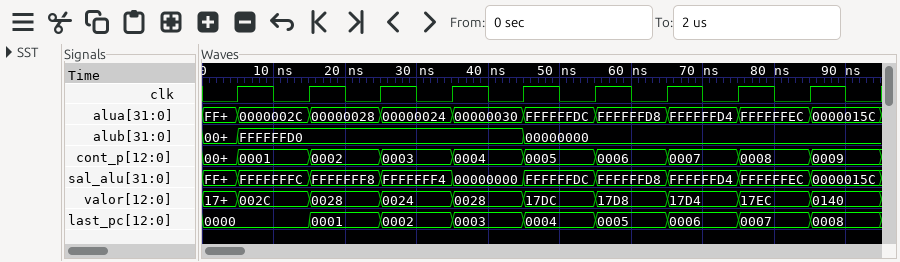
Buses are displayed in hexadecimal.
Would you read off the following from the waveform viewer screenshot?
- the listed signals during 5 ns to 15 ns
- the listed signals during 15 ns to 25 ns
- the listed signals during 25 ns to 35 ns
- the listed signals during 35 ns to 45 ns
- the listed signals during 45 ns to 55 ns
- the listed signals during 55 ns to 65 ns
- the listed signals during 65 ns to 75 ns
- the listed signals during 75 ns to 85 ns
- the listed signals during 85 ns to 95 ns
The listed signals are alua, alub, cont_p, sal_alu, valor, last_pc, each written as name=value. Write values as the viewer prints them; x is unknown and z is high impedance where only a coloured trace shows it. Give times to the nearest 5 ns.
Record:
alua=0000002C, alub=FFFFFFD0, cont_p=0001, sal_alu=FFFFFFFC, valor=002C, last_pc=0000
alua=00000028, alub=FFFFFFD0, cont_p=0002, sal_alu=FFFFFFF8, valor=0028, last_pc=0001
alua=00000024, alub=FFFFFFD0, cont_p=0003, sal_alu=FFFFFFF4, valor=0024, last_pc=0002
alua=00000030, alub=FFFFFFD0, cont_p=0004, sal_alu=00000000, valor=0028, last_pc=0003
alua=FFFFFFDC, alub=00000000, cont_p=0005, sal_alu=FFFFFFDC, valor=17DC, last_pc=0004
alua=FFFFFFD8, alub=00000000, cont_p=0006, sal_alu=FFFFFFD8, valor=17D8, last_pc=0005
alua=FFFFFFD4, alub=00000000, cont_p=0007, sal_alu=FFFFFFD4, valor=17D4, last_pc=0006
alua=FFFFFFEC, alub=00000000, cont_p=0008, sal_alu=FFFFFFEC, valor=17EC, last_pc=0007
alua=0000015C, alub=00000000, cont_p=0009, sal_alu=0000015C, valor=0140, last_pc=0008
